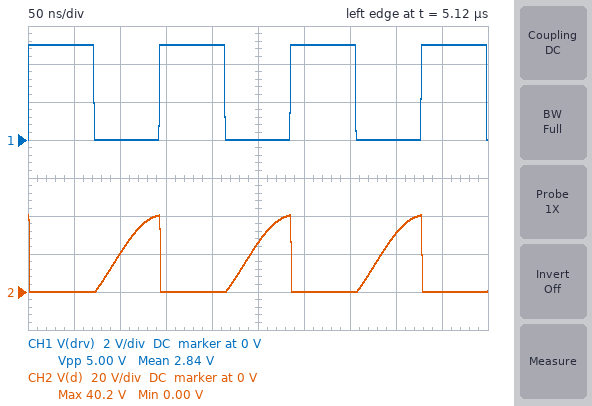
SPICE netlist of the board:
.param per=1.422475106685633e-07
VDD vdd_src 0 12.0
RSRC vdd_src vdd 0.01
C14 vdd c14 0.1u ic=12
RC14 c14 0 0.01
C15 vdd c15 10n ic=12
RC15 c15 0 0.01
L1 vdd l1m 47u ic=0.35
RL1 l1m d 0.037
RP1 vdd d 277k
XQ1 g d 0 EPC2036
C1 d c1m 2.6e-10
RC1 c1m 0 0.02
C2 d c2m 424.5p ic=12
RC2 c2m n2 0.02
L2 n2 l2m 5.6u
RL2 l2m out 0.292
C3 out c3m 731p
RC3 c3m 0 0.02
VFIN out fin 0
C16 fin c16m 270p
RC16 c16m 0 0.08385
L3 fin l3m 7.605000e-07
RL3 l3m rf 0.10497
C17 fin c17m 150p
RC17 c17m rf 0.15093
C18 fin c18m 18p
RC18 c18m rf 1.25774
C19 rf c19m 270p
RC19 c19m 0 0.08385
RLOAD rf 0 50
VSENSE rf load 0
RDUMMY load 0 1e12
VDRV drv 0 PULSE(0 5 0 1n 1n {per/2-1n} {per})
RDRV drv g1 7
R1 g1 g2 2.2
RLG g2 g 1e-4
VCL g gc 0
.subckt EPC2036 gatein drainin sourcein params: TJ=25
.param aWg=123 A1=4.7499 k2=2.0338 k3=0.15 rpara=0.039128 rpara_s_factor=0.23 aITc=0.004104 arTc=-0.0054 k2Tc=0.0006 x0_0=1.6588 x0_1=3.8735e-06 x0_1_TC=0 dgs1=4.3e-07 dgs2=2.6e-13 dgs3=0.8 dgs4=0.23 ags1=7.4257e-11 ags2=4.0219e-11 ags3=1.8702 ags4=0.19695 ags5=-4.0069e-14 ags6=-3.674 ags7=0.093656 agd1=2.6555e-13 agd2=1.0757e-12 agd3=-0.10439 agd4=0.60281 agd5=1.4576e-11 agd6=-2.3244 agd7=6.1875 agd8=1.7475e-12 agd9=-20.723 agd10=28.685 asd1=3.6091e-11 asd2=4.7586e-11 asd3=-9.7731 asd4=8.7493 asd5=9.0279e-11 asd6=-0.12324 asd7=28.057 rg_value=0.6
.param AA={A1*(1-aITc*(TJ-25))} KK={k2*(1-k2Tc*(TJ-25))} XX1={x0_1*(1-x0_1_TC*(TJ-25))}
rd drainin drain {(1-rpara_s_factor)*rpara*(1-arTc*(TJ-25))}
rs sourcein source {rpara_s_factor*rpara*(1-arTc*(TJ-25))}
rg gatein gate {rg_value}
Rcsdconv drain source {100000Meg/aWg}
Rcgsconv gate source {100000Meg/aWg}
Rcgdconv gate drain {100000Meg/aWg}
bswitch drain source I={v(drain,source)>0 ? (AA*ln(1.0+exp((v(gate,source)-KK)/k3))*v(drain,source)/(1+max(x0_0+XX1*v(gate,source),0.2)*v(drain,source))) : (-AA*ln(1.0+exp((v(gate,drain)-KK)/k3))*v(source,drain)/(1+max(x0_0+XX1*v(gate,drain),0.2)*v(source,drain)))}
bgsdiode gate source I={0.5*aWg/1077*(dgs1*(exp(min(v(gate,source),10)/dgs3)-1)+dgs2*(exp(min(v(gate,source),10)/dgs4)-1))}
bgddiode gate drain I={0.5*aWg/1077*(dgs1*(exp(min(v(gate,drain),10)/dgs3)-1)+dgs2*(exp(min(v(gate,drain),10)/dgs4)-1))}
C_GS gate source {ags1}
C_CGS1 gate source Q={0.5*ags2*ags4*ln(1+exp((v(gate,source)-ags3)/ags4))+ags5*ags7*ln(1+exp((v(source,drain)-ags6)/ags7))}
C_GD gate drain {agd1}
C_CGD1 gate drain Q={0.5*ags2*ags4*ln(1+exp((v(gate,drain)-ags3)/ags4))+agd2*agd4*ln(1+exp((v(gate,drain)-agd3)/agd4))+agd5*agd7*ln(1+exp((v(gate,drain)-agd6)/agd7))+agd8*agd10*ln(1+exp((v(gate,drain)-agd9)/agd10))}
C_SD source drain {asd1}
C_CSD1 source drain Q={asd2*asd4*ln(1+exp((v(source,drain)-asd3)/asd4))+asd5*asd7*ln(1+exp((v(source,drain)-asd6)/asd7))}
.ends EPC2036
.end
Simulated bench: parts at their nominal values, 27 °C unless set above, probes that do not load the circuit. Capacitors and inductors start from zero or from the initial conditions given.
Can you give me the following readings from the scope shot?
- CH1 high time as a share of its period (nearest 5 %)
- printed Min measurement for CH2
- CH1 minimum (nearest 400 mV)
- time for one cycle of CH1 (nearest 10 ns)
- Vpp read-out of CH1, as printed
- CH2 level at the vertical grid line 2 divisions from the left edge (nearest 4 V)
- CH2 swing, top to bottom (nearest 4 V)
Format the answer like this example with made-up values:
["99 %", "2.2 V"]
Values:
["50 %", "0.00 V", "0 V", "140 ns", "5.00 V", "20 V", "40 V"]
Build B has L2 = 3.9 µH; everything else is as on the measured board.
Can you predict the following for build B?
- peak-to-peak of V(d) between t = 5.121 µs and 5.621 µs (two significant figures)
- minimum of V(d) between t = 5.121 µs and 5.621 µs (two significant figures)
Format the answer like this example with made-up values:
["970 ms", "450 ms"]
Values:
["35 V", "-4.8 mV"]
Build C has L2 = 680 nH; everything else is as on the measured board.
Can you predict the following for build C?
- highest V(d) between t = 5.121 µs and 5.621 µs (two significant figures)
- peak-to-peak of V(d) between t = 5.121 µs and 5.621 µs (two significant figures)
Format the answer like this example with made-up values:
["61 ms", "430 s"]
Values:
["63 V", "65 V"]
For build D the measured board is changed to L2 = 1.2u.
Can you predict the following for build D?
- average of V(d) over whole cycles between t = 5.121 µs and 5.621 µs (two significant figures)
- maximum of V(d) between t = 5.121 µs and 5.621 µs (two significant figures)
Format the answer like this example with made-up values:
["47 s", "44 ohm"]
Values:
["11 V", "64 V"]
